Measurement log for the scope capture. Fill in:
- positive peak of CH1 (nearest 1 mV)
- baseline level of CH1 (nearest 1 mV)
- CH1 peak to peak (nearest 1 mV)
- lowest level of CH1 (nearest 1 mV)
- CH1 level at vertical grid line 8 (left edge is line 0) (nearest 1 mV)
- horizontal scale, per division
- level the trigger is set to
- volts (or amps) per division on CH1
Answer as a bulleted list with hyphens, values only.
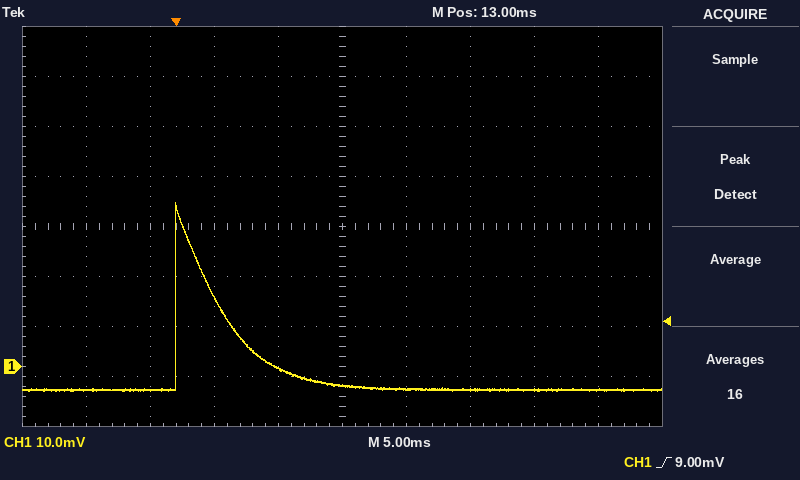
- 33 mV
- -5 mV
- 38 mV
- -5 mV
- -5 mV
- 5 ms
- 9.00 mV
- 10 mV
